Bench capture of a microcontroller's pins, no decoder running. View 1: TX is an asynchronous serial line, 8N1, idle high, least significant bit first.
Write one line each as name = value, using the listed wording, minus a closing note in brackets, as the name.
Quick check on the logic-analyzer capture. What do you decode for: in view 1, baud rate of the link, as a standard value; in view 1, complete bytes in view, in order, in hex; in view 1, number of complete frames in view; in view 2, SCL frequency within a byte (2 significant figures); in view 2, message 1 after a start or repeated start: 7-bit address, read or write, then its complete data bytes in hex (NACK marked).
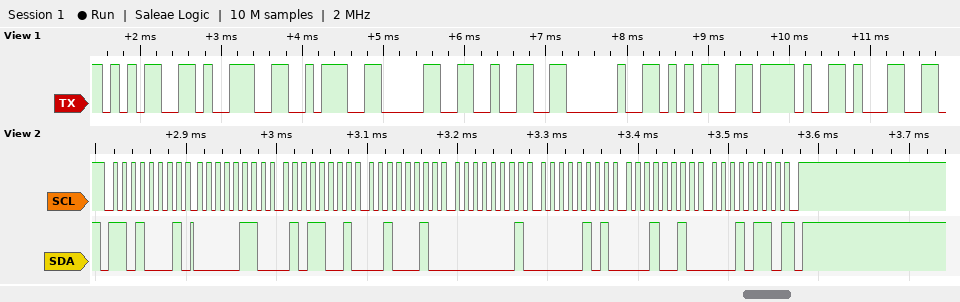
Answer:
in view 1, baud rate of the link, as a standard value = 9600 baud
in view 1, complete bytes in view, in order, in hex = 35 39 3A 30 32 20 35 2F 31
in view 1, number of complete frames in view = 9
in view 2, SCL frequency within a byte = 100 kHz
in view 2, message 1 after a start or repeated start: 7-bit address, read or write, then its complete data bytes in hex = 0x68 read: 06 59 22 01 05 12 16 NACK
